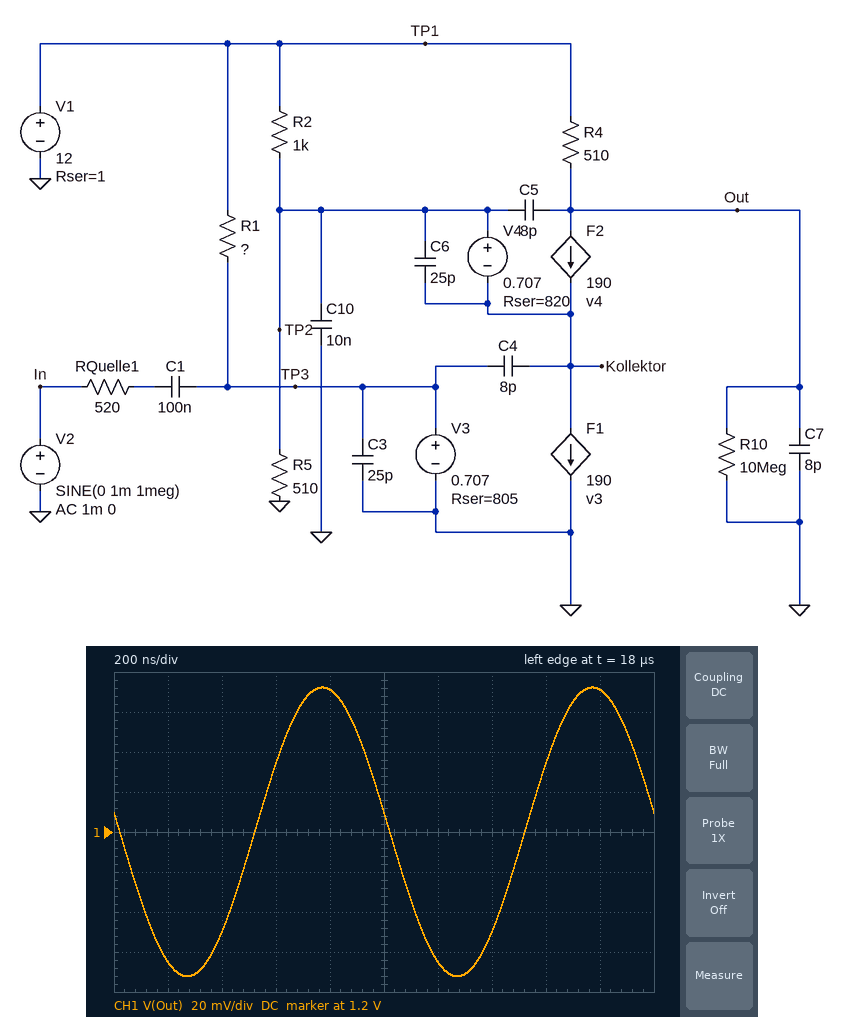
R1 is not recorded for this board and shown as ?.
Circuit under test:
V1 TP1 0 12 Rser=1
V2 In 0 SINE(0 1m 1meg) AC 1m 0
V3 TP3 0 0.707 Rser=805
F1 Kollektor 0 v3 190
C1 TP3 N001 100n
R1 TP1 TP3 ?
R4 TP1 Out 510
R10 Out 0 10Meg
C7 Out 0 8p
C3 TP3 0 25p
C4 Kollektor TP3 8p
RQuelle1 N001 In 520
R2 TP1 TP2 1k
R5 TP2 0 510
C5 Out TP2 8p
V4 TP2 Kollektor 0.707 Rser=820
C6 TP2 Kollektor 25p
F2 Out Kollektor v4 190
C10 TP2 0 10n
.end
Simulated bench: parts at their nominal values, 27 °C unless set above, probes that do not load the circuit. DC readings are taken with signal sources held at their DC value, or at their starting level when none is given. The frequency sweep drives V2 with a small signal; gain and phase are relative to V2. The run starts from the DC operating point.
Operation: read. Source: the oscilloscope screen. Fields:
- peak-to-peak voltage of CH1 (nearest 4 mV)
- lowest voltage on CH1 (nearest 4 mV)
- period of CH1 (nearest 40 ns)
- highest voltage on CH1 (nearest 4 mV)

144 mV
1.128 V
1.00 µs
1.272 V
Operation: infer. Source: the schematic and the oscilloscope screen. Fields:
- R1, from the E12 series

100 kΩ
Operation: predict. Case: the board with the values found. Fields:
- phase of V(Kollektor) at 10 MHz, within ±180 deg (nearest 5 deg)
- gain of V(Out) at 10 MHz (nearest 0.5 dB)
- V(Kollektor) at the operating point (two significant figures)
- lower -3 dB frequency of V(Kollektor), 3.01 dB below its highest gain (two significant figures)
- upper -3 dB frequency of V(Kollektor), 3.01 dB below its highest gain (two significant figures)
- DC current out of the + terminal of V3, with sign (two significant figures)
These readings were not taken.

140 deg
34.0 dB
3.2 V
1.2 kHz
4.0 MHz
-110 µA
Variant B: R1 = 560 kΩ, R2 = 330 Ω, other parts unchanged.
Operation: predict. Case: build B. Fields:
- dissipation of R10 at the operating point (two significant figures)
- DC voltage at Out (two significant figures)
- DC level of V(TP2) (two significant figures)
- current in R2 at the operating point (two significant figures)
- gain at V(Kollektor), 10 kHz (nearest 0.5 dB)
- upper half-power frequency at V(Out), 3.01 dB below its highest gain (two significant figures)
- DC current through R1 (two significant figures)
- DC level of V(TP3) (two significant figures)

10 µW
10 V
7.3 V
14 mA
-1.5 dB
9.4 MHz
20 µA
720 mV
